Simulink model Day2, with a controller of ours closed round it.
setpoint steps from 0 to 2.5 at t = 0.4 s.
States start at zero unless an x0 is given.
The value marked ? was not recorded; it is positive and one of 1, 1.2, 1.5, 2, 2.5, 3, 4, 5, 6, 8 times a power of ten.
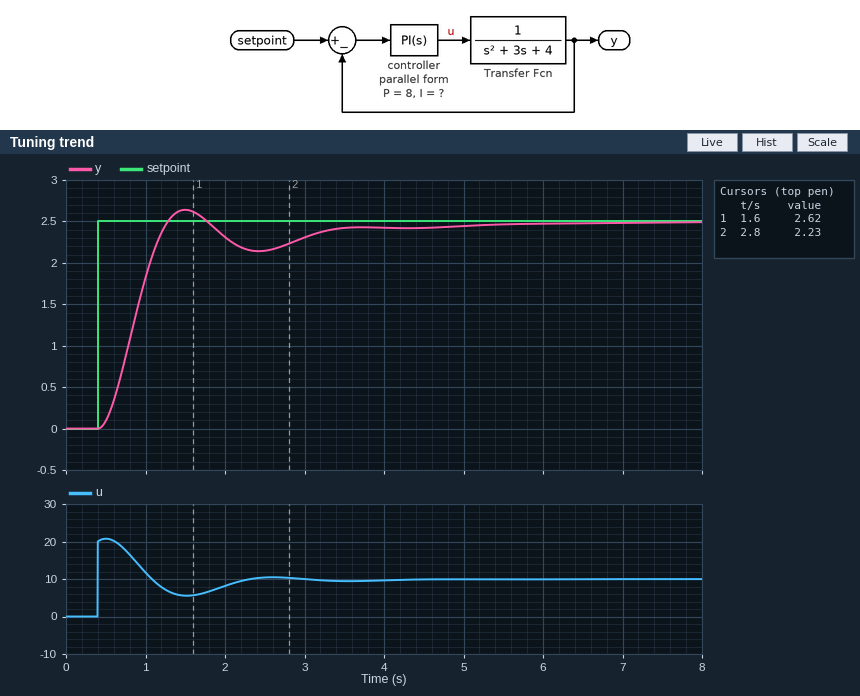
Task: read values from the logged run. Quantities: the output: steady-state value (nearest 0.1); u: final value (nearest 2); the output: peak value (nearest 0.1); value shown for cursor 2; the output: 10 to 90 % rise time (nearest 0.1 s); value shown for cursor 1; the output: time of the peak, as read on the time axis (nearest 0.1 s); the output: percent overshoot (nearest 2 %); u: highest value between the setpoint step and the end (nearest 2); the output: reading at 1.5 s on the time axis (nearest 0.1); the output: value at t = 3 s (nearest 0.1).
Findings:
2.5
10
2.6
2.23
0.6 s
2.62
1.5 s
6 %
20
2.6
2.3
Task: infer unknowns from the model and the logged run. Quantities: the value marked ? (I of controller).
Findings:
6
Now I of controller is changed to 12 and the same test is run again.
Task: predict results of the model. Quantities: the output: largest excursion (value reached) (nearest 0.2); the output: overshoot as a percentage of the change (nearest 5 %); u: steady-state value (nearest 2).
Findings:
3.2
25 %
10
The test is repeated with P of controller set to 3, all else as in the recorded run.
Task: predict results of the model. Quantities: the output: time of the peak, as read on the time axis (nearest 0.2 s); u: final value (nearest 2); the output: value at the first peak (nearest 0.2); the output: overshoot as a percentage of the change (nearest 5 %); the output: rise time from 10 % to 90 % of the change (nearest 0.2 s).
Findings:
2.2 s
10
2.8
10 %
0.8 s
